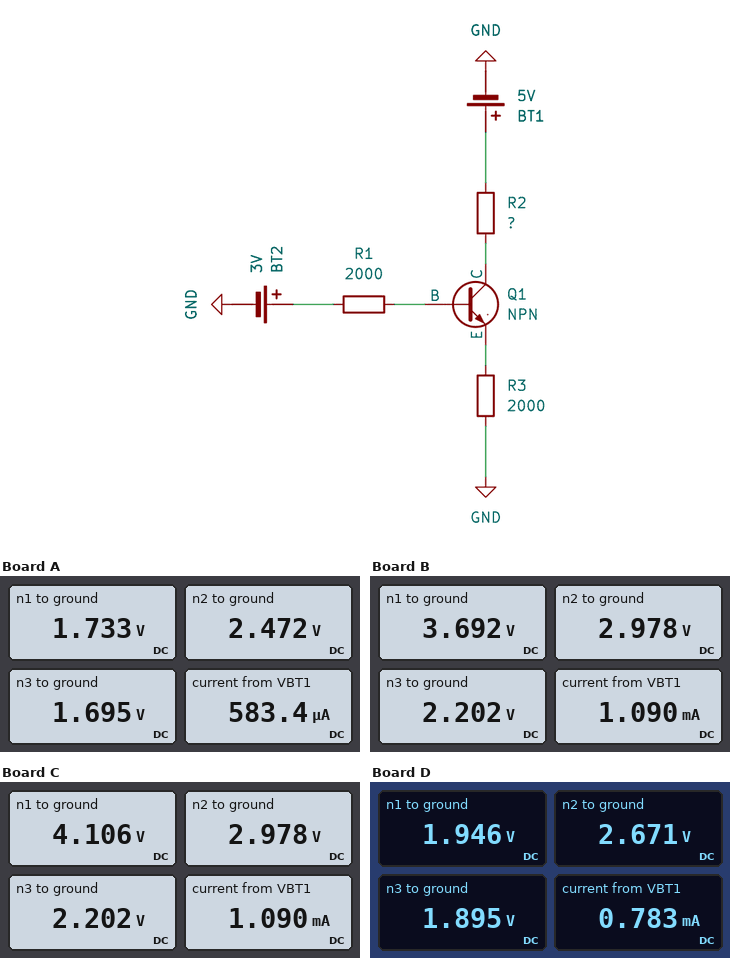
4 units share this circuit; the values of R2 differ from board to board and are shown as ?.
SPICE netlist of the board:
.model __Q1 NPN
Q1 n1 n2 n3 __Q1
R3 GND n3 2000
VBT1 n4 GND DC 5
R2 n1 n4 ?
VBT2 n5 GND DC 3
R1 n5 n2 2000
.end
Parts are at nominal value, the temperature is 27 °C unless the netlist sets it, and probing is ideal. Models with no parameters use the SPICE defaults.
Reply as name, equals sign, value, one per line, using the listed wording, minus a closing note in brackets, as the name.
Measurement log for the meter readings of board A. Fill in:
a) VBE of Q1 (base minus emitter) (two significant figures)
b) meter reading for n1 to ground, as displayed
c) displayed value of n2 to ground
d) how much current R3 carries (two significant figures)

VBE of Q1 (base minus emitter) = 780 mV
meter reading for n1 to ground, as displayed = 1.733 V
displayed value of n2 to ground = 2.472 V
how much current R3 carries = 850 µA
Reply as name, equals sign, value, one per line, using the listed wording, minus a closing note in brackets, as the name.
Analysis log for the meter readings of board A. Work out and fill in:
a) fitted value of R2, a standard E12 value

fitted value of R2, a standard E12 value = 5.6 kΩ
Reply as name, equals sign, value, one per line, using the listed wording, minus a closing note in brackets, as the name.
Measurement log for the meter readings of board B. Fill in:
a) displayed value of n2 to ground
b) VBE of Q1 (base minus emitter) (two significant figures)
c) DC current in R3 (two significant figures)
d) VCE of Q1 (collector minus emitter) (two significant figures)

displayed value of n2 to ground = 2.978 V
VBE of Q1 (base minus emitter) = 780 mV
DC current in R3 = 1.1 mA
VCE of Q1 (collector minus emitter) = 1.5 V
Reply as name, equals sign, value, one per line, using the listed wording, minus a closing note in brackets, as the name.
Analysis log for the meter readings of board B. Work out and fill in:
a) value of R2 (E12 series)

value of R2 = 1.2 kΩ
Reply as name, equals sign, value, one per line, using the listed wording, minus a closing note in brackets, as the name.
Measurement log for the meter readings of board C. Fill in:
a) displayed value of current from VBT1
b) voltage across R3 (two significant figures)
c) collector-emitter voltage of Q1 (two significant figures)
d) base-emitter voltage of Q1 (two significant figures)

displayed value of current from VBT1 = 1.090 mA
voltage across R3 = 2.2 V
collector-emitter voltage of Q1 = 1.9 V
base-emitter voltage of Q1 = 780 mV
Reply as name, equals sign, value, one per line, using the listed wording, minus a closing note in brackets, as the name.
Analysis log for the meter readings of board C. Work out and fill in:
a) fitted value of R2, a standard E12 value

fitted value of R2, a standard E12 value = 820 Ω
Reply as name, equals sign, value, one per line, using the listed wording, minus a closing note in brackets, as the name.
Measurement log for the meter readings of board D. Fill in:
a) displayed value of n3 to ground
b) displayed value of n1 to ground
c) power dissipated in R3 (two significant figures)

displayed value of n3 to ground = 1.895 V
displayed value of n1 to ground = 1.946 V
power dissipated in R3 = 1.8 mW
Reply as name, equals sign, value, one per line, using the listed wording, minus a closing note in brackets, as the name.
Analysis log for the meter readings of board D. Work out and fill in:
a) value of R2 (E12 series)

value of R2 = 3.9 kΩ
